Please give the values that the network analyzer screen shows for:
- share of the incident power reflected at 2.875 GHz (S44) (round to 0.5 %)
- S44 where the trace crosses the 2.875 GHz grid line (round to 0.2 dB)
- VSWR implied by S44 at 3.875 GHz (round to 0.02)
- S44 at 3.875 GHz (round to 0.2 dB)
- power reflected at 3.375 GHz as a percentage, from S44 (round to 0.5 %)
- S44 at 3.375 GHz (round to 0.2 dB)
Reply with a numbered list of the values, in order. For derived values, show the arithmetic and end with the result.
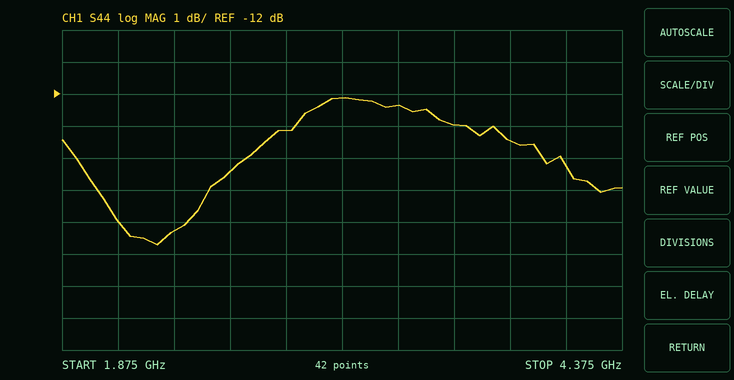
1. 10^(-13.2/10) ≈ 4.79 %, so 5.0 % to the nearest 0.5 %
2. -13.2 dB
3. |Γ| = 10^(-13.4/20) = 0.2138; VSWR = (1 + 0.2138)/(1 − 0.2138) ≈ 1.54
4. -13.4 dB
5. 10^(-12.4/10) ≈ 5.75 %, so 6.0 % to the nearest 0.5 %
6. -12.4 dB
